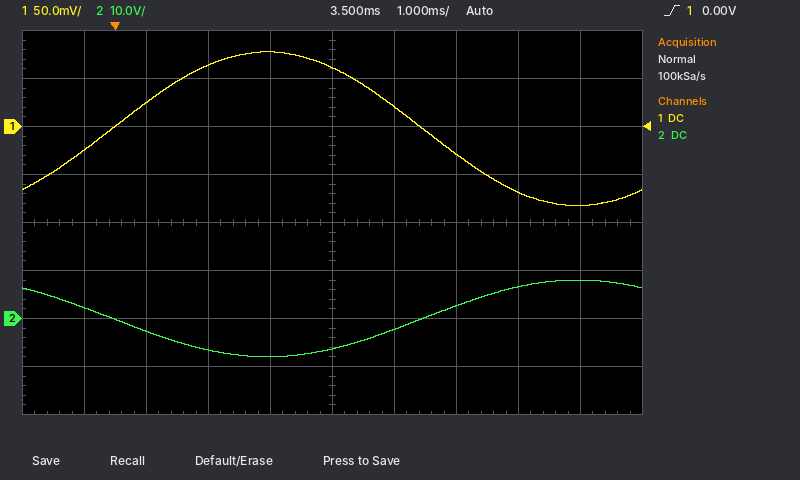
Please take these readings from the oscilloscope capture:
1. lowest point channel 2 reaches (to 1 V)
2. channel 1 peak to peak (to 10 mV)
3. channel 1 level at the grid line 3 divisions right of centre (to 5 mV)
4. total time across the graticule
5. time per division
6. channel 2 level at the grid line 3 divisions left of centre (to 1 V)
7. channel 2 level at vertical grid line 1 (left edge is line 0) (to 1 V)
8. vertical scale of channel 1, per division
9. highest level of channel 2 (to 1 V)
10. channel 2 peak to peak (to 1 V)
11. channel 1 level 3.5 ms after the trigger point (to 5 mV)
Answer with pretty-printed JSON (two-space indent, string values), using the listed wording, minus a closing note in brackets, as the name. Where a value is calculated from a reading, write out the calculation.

{
  "lowest point channel 2 reaches": "-8 V",
  "channel 1 peak to peak": "160 mV",
  "channel 1 level at the grid line 3 divisions right of centre": "-70 mV",
  "total time across the graticule": "10 ms",
  "time per division": "1 ms",
  "channel 2 level at the grid line 3 divisions left of centre": "-3 V",
  "channel 2 level at vertical grid line 1 (left edge is line 0)": "2 V",
  "vertical scale of channel 1, per division": "50 mV",
  "highest level of channel 2": "8 V",
  "channel 2 peak to peak": "8 V − (-8 V) = 16 V",
  "channel 1 level 3.5 ms after the trigger point": "60 mV"
}
